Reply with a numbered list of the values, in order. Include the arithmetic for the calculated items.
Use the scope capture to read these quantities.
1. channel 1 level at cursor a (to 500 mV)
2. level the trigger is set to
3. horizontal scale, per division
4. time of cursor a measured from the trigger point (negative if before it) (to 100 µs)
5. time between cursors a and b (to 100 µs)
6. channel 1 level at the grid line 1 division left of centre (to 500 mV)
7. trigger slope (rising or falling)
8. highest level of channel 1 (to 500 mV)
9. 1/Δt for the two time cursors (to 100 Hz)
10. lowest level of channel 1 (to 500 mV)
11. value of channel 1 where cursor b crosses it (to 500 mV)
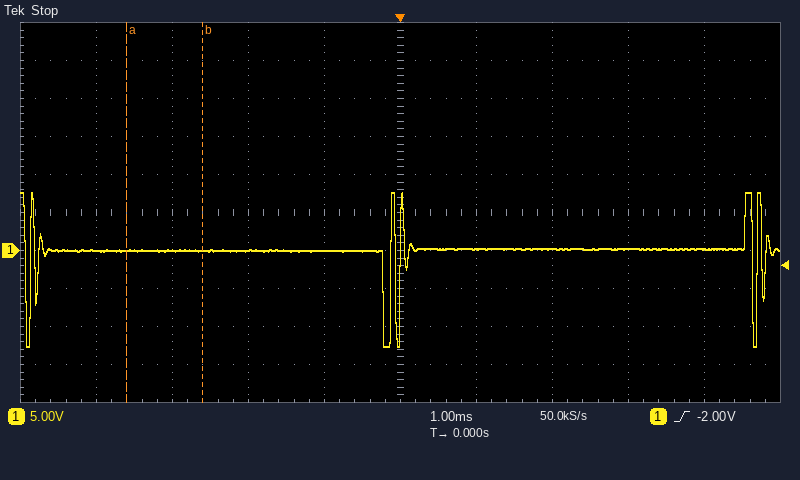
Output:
1. 0.0 V
2. -2.00 V
3. 1 ms
4. -3.6 ms
5. 1.0 ms
6. 0.0 V
7. rising
8. 7.5 V
9. 1 / 1.0 ms ≈ 1.0 kHz
10. -12.5 V
11. 0.0 V
